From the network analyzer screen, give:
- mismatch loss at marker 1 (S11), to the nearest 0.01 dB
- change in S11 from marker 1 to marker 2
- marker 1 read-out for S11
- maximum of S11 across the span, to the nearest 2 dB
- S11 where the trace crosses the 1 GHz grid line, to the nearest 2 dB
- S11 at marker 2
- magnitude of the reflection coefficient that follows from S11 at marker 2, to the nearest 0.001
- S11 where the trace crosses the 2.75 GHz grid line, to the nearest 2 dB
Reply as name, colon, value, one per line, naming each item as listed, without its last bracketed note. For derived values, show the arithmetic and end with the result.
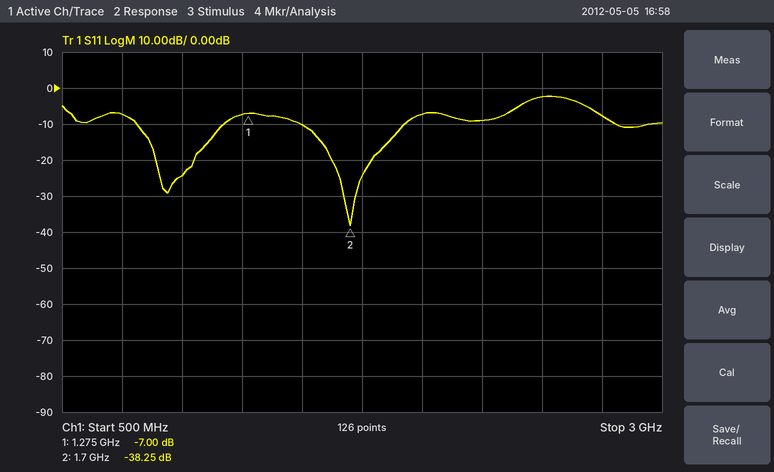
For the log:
mismatch loss at marker 1 (S11), to the nearest 0.01 dB: −10 log10(1 − 10^(-7/10)) ≈ 0.97 dB
change in S11 from marker 1 to marker 2: -38.25 − (-7) = -31.25 dB
marker 1 read-out for S11: -7.00 dB
maximum of S11 across the span, to the nearest 2 dB: -2 dB
S11 where the trace crosses the 1 GHz grid line, to the nearest 2 dB: -24 dB
S11 at marker 2: -38.25 dB
magnitude of the reflection coefficient that follows from S11 at marker 2, to the nearest 0.001: 10^(-38.25/20) ≈ 0.012
S11 where the trace crosses the 2.75 GHz grid line, to the nearest 2 dB: -8 dB
